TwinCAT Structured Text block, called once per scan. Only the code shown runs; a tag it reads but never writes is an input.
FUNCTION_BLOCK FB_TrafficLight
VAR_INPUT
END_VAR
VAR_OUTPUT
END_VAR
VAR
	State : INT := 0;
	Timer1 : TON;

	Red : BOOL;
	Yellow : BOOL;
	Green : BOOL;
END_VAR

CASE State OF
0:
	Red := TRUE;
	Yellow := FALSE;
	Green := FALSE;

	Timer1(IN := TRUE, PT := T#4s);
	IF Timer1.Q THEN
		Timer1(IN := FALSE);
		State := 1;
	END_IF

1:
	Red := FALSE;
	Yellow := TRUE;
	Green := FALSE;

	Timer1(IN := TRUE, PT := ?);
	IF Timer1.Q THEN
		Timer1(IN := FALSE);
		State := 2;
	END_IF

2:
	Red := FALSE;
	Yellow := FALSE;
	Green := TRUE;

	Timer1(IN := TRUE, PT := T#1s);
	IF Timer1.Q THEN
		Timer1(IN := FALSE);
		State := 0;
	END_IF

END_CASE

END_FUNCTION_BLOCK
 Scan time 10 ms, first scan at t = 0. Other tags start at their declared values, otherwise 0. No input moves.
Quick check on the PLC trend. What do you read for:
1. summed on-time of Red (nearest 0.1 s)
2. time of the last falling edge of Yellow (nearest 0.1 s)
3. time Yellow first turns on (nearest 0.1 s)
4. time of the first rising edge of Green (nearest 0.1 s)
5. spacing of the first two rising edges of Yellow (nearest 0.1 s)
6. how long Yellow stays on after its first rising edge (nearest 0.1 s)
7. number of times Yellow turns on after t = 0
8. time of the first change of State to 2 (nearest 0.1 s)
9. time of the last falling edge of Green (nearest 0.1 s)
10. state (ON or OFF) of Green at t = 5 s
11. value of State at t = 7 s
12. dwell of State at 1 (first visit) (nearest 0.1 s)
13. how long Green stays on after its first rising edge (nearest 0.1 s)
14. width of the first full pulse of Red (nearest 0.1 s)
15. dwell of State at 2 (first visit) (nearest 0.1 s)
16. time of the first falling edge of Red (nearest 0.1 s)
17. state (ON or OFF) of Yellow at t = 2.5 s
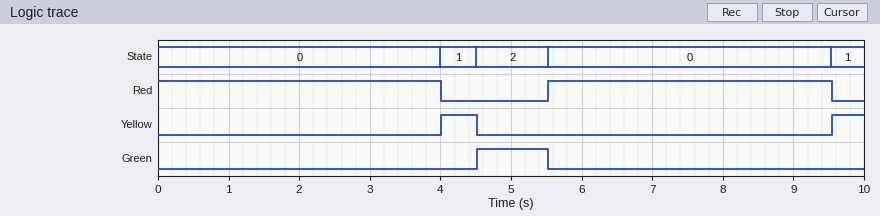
8.0 s
4.5 s
4.0 s
4.5 s
5.5 s
0.5 s
2
4.5 s
5.5 s
ON
0
0.5 s
1.0 s
4.0 s
1.0 s
4.0 s
OFF
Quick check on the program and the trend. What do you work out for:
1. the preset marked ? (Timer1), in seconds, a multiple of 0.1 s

0.5 s
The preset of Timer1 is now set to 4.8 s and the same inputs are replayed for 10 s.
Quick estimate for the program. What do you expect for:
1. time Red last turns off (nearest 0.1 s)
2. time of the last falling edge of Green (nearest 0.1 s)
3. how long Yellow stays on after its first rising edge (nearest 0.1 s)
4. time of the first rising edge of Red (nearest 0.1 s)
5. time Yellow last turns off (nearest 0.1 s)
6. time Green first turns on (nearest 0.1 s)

4.0 s
9.8 s
4.8 s
9.8 s
8.8 s
8.8 s
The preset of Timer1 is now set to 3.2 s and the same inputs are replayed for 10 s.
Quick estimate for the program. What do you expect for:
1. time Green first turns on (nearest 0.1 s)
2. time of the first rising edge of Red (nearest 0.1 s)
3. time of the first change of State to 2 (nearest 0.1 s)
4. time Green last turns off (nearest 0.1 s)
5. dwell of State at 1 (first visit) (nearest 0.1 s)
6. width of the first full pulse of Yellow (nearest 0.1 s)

7.2 s
8.2 s
7.2 s
8.2 s
3.2 s
3.2 s
